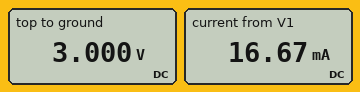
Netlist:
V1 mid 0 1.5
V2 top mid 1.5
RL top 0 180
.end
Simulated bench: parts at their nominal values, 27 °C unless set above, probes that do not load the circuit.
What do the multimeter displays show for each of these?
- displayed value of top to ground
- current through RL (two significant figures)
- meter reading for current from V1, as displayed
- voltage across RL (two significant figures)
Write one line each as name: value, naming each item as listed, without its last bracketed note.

displayed value of top to ground: 3.000 V
current through RL: 17 mA
meter reading for current from V1, as displayed: 16.67 mA
voltage across RL: 3.0 V
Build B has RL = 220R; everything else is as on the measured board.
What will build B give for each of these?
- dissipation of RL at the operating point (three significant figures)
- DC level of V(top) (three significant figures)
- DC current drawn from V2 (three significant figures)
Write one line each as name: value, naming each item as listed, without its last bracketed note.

dissipation of RL at the operating point: 40.9 mW
DC level of V(top): 3.00 V
DC current drawn from V2: 13.6 mA
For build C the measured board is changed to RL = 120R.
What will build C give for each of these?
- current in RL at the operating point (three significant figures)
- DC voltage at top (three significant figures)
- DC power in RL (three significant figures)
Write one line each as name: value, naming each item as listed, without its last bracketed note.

current in RL at the operating point: 25.0 mA
DC voltage at top: 3.00 V
DC power in RL: 75.0 mW
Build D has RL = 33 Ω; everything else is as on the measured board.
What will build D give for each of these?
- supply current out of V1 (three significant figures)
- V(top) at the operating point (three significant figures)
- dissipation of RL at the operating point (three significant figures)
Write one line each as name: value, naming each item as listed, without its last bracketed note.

supply current out of V1: 90.9 mA
V(top) at the operating point: 3.00 V
dissipation of RL at the operating point: 273 mW
